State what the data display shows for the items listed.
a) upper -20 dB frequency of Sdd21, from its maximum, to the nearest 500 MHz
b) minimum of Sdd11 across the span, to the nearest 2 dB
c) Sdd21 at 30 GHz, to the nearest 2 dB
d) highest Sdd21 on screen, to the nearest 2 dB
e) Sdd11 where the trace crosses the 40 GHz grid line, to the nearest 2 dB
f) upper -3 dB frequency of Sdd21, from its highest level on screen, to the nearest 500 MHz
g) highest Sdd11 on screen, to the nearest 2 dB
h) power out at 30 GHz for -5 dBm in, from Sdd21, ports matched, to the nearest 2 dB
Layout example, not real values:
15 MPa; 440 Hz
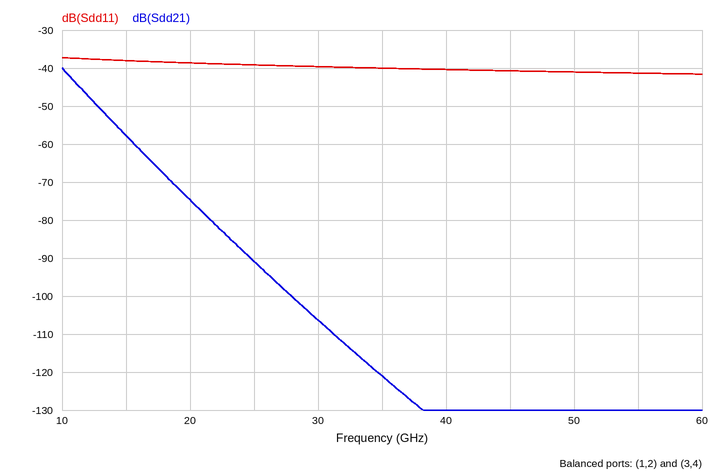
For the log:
15.5 GHz; -42 dB; -106 dB; -40 dB; -40 dB; 11.0 GHz; -38 dB; -112 dBm
